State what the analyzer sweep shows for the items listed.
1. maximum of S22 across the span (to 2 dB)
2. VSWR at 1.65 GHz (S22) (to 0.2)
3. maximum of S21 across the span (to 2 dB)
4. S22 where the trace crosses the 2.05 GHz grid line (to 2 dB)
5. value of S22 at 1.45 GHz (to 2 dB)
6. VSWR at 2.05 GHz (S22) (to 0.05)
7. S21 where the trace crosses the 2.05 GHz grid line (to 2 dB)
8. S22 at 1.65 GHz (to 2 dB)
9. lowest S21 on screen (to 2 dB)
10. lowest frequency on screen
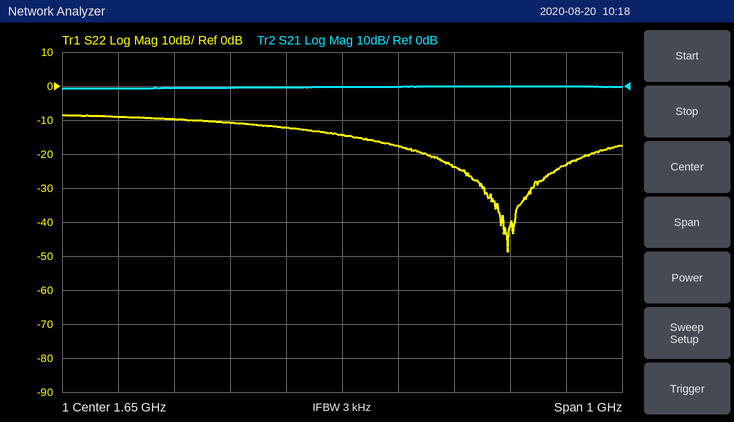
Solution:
-8 dB
1.4
0 dB
-24 dB
-10 dB
1.15
0 dB
-14 dB
0 dB
1.15 GHz
